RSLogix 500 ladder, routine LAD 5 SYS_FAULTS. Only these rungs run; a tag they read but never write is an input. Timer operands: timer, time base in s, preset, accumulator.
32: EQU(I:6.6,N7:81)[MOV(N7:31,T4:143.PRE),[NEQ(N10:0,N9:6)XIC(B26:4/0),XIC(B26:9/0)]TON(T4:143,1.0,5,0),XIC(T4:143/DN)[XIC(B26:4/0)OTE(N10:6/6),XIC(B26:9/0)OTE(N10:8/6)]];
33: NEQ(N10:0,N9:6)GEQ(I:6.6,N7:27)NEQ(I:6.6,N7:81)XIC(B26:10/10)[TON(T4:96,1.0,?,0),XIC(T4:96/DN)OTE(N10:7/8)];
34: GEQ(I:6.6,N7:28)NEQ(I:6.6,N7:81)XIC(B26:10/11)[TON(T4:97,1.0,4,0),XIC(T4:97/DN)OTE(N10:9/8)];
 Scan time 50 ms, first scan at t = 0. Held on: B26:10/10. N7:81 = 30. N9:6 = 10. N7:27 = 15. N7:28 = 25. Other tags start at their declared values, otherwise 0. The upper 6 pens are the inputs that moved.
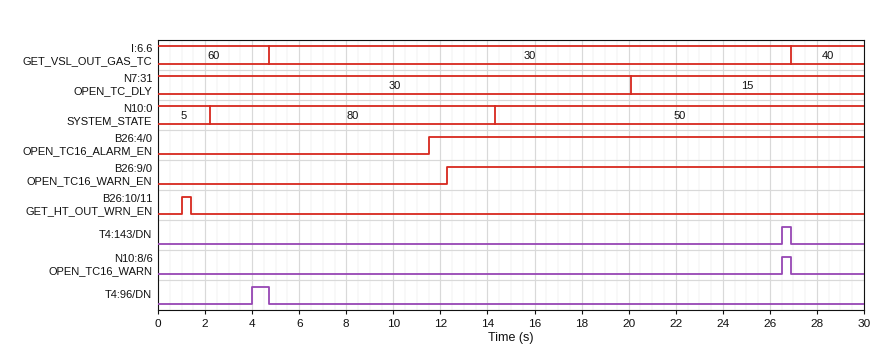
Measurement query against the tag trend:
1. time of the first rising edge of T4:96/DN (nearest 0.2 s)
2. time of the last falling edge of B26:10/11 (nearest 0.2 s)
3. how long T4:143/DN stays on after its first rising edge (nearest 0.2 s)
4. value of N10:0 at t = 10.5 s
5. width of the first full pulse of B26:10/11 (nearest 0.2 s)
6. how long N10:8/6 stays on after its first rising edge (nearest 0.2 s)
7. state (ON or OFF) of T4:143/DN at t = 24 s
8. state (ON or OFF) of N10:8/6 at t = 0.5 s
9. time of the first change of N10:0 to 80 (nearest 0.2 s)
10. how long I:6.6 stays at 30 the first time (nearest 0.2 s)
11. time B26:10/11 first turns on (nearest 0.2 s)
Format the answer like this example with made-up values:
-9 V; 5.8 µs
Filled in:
4.0 s; 1.4 s; 0.4 s; 80; 0.4 s; 0.4 s; OFF; OFF; 2.2 s; 22.2 s; 1.0 s
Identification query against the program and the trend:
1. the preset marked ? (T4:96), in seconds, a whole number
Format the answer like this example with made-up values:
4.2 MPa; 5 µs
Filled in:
4 s
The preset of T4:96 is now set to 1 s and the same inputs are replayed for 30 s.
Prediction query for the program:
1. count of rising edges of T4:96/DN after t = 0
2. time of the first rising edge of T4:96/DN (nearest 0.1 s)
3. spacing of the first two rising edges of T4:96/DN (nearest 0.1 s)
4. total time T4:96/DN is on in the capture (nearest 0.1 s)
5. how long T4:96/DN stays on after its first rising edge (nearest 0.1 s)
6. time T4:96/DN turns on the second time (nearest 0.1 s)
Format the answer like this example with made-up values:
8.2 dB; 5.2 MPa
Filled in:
2; 1.0 s; 26.9 s; 5.8 s; 3.7 s; 27.9 s
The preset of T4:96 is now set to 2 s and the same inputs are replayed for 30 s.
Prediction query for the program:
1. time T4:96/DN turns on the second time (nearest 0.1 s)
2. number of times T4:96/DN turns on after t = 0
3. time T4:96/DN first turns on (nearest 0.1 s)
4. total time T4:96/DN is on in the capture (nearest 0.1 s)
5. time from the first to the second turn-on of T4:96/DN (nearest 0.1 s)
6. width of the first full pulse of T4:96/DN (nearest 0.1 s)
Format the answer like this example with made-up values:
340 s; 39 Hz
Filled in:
28.9 s; 2; 2.0 s; 3.8 s; 26.9 s; 2.7 s
